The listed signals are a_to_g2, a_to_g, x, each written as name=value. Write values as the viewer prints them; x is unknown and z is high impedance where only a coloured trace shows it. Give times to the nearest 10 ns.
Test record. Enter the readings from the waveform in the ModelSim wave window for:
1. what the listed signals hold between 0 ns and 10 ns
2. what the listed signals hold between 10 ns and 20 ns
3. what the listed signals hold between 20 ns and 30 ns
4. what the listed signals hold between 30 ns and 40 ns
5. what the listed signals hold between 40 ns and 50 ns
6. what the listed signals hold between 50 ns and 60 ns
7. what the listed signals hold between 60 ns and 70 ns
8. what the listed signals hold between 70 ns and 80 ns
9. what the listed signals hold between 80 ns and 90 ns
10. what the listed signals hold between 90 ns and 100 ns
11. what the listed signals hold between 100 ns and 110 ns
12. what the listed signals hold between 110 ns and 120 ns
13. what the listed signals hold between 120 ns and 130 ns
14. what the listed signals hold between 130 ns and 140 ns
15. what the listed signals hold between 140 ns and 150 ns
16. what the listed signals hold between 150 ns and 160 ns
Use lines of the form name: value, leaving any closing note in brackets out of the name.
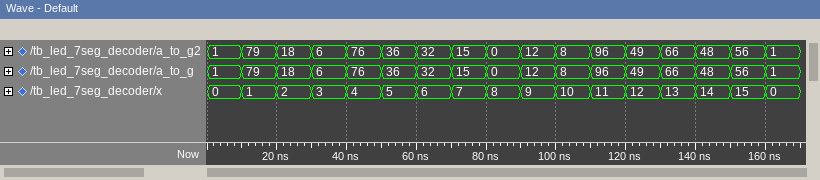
what the listed signals hold between 0 ns and 10 ns: a_to_g2=1, a_to_g=1, x=0
what the listed signals hold between 10 ns and 20 ns: a_to_g2=79, a_to_g=79, x=1
what the listed signals hold between 20 ns and 30 ns: a_to_g2=18, a_to_g=18, x=2
what the listed signals hold between 30 ns and 40 ns: a_to_g2=6, a_to_g=6, x=3
what the listed signals hold between 40 ns and 50 ns: a_to_g2=76, a_to_g=76, x=4
what the listed signals hold between 50 ns and 60 ns: a_to_g2=36, a_to_g=36, x=5
what the listed signals hold between 60 ns and 70 ns: a_to_g2=32, a_to_g=32, x=6
what the listed signals hold between 70 ns and 80 ns: a_to_g2=15, a_to_g=15, x=7
what the listed signals hold between 80 ns and 90 ns: a_to_g2=0, a_to_g=0, x=8
what the listed signals hold between 90 ns and 100 ns: a_to_g2=12, a_to_g=12, x=9
what the listed signals hold between 100 ns and 110 ns: a_to_g2=8, a_to_g=8, x=10
what the listed signals hold between 110 ns and 120 ns: a_to_g2=96, a_to_g=96, x=11
what the listed signals hold between 120 ns and 130 ns: a_to_g2=49, a_to_g=49, x=12
what the listed signals hold between 130 ns and 140 ns: a_to_g2=66, a_to_g=66, x=13
what the listed signals hold between 140 ns and 150 ns: a_to_g2=48, a_to_g=48, x=14
what the listed signals hold between 150 ns and 160 ns: a_to_g2=56, a_to_g=56, x=15
